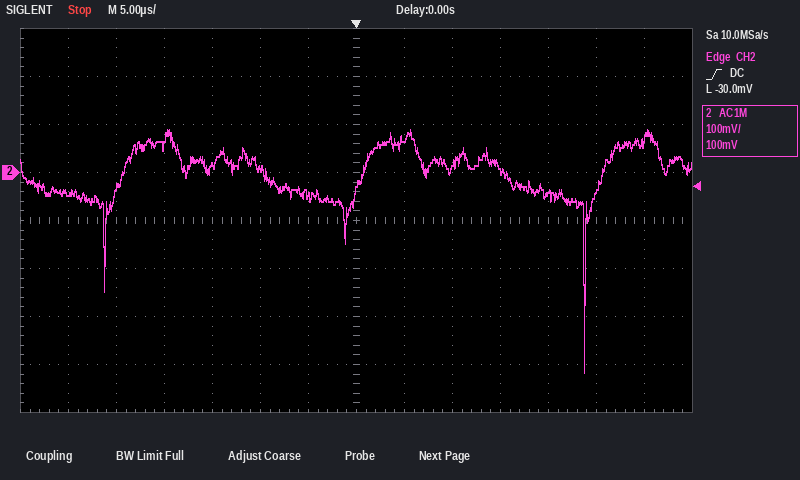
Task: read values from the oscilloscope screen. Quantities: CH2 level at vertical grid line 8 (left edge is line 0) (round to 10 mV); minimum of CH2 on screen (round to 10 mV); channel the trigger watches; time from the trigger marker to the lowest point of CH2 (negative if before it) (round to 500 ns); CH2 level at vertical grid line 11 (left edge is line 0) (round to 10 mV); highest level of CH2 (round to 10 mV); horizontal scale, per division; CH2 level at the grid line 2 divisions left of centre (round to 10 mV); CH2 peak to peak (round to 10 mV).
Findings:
70 mV
-420 mV
CH2
+24.0 µs
-40 mV
90 mV
5 µs
10 mV
510 mV
